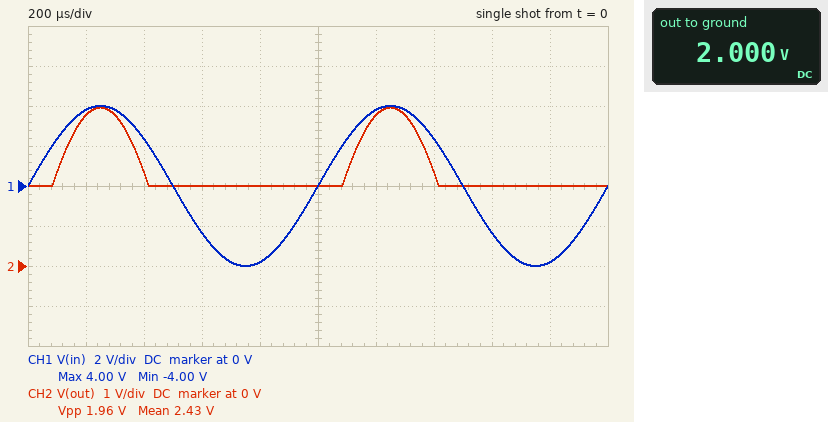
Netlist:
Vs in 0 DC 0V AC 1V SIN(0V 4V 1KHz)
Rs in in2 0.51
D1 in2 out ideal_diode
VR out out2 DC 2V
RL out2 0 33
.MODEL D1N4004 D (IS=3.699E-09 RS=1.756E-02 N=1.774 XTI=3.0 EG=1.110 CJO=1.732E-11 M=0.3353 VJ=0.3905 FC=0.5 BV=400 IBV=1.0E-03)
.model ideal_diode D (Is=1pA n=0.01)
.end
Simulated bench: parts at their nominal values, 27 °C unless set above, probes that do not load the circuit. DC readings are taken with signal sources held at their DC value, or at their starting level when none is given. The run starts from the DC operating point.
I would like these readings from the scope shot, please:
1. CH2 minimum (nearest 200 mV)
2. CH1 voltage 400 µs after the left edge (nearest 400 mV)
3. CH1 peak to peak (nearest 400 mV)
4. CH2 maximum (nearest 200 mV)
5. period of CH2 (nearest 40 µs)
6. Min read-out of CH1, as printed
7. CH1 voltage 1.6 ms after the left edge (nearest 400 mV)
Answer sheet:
2.0 V
2.4 V
8.0 V
4.0 V
1.00 ms
-4.00 V
-2.4 V
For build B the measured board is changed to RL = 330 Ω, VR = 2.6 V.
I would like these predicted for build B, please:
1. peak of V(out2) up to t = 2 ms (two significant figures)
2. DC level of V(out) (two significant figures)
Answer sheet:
1.4 V
2.6 V
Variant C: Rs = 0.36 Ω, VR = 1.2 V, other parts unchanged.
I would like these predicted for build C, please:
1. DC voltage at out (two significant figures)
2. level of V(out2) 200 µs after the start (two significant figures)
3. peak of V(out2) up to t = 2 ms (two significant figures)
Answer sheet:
1.2 V
2.6 V
2.8 V
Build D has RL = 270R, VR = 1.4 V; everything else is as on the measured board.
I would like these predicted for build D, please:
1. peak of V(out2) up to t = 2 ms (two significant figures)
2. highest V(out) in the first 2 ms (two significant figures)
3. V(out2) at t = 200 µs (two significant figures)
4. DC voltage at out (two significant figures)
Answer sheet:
2.6 V
4.0 V
2.4 V
1.4 V
